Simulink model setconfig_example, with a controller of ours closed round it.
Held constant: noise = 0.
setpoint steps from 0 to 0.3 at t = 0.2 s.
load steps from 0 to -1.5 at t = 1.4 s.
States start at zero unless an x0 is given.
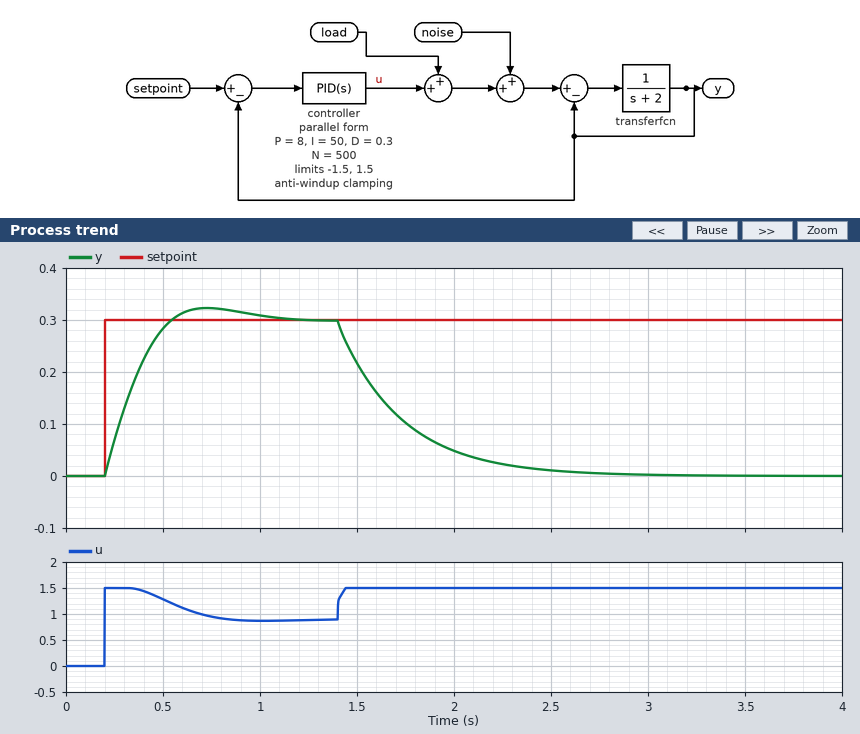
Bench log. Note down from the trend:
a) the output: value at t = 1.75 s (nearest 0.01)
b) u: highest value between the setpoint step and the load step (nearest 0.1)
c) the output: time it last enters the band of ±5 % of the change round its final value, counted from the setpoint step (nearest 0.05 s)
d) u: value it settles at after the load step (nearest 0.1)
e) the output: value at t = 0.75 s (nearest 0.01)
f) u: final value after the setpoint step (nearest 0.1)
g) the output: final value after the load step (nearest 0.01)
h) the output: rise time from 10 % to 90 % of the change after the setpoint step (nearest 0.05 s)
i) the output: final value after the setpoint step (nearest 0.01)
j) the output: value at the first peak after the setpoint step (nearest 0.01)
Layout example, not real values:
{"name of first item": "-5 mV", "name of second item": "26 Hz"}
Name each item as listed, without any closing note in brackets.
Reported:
{"the output: value at t = 1.75 s": "0.10", "u: highest value between the setpoint step and the load step": "1.5", "the output: time it last enters the band of ±5 % of the change round its final value, counted from the setpoint step": "0.70 s", "u: value it settles at after the load step": "1.5", "the output: value at t = 0.75 s": "0.32", "u: final value after the setpoint step": "0.9", "the output: final value after the load step": "0.00", "the output: rise time from 10 % to 90 % of the change after the setpoint step": "0.25 s", "the output: final value after the setpoint step": "0.30", "the output: value at the first peak after the setpoint step": "0.32"}
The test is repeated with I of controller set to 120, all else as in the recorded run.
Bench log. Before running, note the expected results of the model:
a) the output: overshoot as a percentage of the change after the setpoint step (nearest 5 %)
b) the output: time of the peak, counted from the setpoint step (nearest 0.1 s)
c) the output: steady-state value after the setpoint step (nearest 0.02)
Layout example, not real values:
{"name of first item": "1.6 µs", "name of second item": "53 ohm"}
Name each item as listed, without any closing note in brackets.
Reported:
{"the output: overshoot as a percentage of the change after the setpoint step": "10 %", "the output: time of the peak, counted from the setpoint step": "0.4 s", "the output: steady-state value after the setpoint step": "0.30"}
